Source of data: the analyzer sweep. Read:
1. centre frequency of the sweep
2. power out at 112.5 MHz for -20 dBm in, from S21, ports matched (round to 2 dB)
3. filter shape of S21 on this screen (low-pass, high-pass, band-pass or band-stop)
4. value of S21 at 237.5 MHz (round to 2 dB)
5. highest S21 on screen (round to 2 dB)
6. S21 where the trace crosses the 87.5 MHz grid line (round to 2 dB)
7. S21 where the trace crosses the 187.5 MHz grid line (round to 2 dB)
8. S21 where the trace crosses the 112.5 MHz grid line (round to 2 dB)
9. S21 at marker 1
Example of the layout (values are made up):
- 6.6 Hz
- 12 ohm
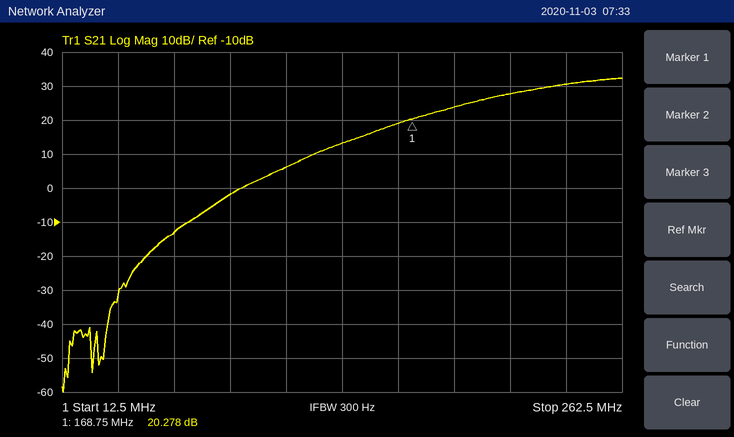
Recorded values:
- 137.5 MHz
- -14 dBm
- high-pass
- 30 dB
- 32 dB
- -2 dB
- 24 dB
- 6 dB
- 20.278 dB
